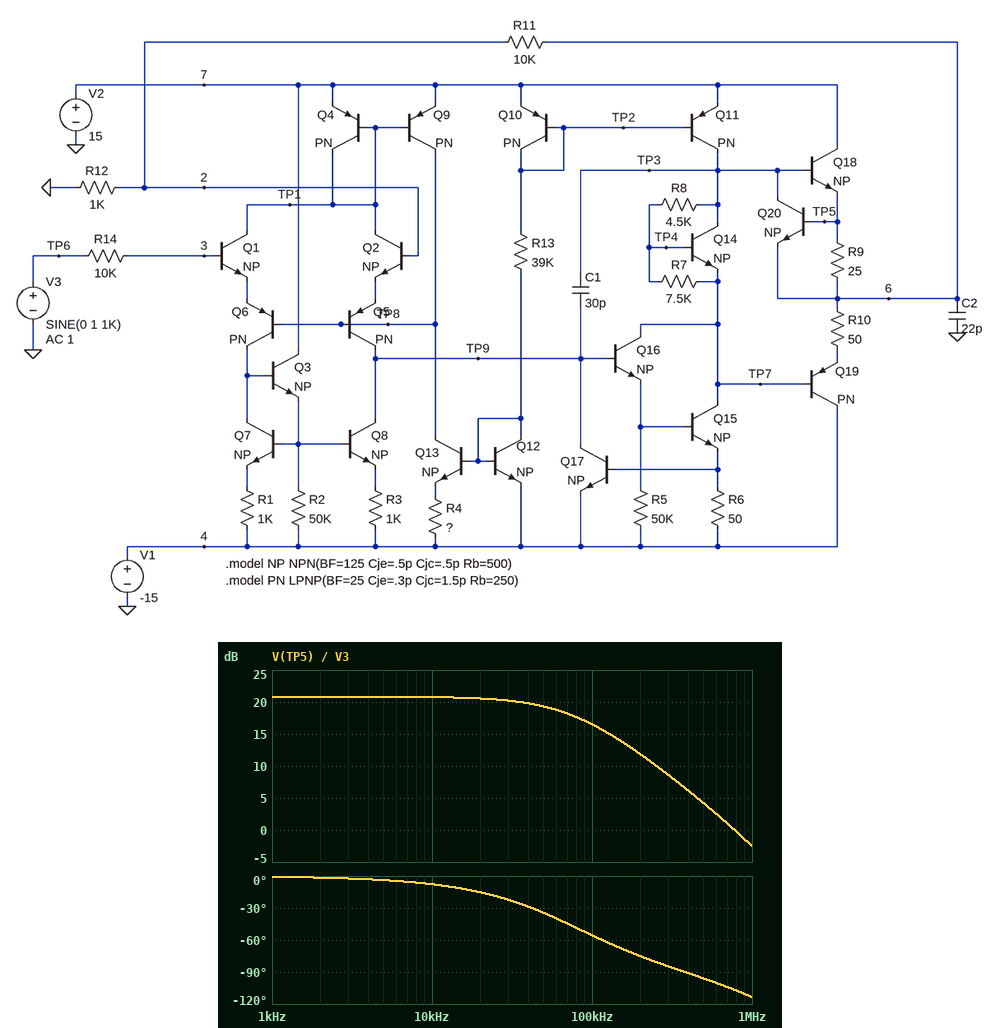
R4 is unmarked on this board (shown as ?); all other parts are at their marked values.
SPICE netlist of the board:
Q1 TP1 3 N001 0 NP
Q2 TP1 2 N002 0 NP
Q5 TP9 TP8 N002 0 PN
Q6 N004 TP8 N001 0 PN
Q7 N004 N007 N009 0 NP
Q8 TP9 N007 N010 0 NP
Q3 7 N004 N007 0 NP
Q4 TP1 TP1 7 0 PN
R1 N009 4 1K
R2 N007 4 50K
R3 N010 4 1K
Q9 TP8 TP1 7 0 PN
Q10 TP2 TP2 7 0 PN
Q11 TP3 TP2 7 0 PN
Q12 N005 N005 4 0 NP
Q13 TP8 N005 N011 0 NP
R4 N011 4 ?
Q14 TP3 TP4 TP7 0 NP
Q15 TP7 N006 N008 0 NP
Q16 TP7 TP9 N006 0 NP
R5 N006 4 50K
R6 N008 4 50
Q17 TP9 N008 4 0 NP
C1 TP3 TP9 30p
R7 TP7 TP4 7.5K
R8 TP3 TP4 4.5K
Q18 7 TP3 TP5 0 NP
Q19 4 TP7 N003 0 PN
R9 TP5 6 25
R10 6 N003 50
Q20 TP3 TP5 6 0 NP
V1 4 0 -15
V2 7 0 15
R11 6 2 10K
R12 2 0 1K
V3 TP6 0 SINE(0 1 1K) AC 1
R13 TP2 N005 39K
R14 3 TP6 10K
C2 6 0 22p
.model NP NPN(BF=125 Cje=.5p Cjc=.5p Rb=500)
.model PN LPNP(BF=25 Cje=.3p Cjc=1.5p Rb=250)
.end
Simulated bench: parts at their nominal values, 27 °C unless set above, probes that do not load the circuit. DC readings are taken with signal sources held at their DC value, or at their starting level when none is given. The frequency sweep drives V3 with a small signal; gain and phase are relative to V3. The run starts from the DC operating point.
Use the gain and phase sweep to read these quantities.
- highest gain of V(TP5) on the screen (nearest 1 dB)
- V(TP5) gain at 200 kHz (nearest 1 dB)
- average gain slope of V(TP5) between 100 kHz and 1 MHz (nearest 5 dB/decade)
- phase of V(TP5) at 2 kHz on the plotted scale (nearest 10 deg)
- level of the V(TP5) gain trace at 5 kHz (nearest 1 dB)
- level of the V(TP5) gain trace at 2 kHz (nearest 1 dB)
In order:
21 dB
12 dB
-20 dB/decade
0 deg
21 dB
21 dB
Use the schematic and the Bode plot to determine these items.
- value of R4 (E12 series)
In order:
3.9 kΩ
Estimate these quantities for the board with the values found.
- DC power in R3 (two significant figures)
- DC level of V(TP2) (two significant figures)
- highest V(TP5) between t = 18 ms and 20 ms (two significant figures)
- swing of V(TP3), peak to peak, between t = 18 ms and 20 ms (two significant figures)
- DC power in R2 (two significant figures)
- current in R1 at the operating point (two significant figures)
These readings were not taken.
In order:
140 nW
14 V
11 V
22 V
9.0 µW
12 µA
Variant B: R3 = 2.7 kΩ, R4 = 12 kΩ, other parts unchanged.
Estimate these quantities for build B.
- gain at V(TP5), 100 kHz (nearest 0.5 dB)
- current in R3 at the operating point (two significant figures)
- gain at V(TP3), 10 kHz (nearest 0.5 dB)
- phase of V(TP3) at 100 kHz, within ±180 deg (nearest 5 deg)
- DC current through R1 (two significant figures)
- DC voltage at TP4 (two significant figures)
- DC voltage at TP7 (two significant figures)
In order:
10.0 dB
4.1 µA
22.0 dB
-75 deg
5.2 µA
-21 mV
-780 mV
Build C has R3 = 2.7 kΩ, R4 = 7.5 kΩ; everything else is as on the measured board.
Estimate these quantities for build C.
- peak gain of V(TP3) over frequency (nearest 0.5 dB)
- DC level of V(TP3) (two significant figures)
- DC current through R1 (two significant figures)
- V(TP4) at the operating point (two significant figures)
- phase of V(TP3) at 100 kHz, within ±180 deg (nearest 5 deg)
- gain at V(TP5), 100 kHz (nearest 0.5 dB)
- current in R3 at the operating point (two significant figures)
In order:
22.0 dB
400 mV
7.9 µA
-77 mV
-65 deg
13.0 dB
5.9 µA
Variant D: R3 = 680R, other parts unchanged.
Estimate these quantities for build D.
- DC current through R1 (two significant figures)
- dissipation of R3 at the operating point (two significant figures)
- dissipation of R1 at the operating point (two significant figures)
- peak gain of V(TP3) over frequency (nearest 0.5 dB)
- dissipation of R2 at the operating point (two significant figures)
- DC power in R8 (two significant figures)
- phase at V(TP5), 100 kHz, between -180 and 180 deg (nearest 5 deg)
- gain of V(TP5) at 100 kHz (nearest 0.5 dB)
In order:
11 µA
100 nW
120 nW
23.5 dB
8.9 µW
51 µW
-50 deg
17.5 dB
